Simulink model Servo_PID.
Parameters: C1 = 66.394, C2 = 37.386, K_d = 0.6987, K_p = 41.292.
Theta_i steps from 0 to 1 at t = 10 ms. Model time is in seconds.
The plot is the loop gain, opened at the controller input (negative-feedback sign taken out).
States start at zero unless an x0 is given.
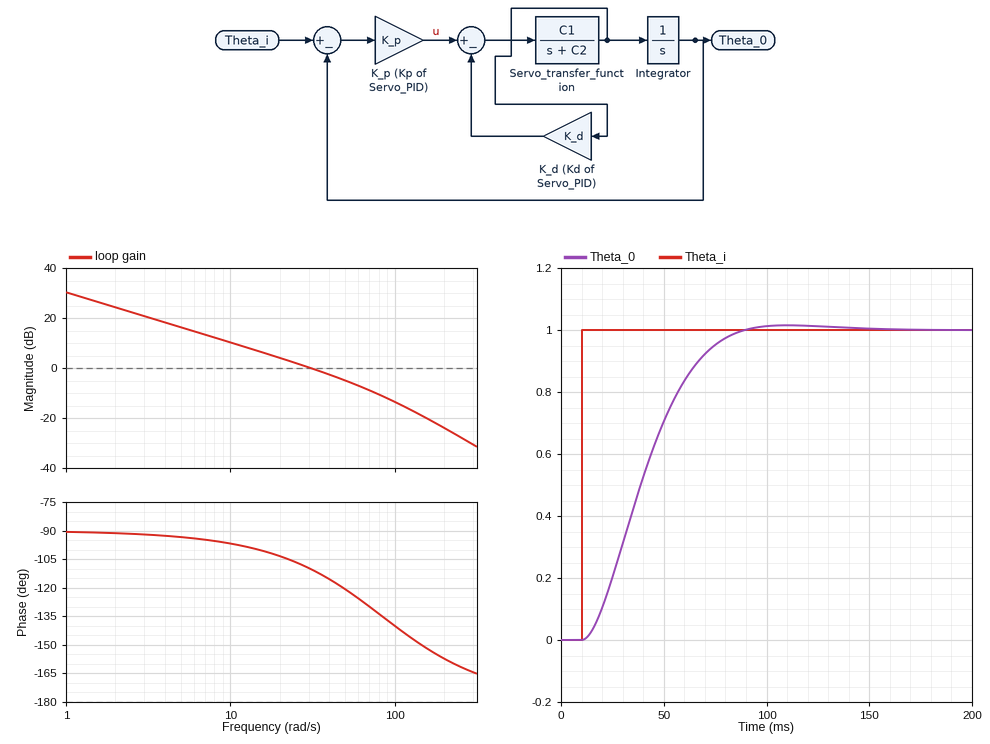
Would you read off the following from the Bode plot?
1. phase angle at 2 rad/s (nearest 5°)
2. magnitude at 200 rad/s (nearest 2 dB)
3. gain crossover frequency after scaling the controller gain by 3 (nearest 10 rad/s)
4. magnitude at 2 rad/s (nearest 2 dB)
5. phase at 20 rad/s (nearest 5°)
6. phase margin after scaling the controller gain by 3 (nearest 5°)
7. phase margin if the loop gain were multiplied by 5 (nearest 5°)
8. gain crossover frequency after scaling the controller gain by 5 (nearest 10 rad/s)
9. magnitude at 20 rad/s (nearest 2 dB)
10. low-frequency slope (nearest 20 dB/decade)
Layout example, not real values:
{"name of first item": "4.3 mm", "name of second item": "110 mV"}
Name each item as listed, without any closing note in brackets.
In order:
{"phase angle at 2 rad/s": "-90°", "magnitude at 200 rad/s": "-24 dB", "gain crossover frequency after scaling the controller gain by 3": "70 rad/s", "magnitude at 2 rad/s": "24 dB", "phase at 20 rad/s": "-105°", "phase margin after scaling the controller gain by 3": "50°", "phase margin if the loop gain were multiplied by 5": "40°", "gain crossover frequency after scaling the controller gain by 5": "100 rad/s", "magnitude at 20 rad/s": "4 dB", "low-frequency slope": "-20 dB/decade"}
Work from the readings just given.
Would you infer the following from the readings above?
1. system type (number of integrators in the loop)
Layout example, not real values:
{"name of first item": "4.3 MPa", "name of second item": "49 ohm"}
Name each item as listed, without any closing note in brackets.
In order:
{"system type": "1"}
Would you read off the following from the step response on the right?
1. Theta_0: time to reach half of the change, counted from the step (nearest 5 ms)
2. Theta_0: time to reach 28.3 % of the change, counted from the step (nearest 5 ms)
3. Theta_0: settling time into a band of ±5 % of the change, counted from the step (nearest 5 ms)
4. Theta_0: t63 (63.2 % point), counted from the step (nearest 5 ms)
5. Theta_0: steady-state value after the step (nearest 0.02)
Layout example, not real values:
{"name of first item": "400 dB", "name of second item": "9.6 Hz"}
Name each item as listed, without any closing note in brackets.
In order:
{"Theta_0: time to reach half of the change, counted from the step": "30 ms", "Theta_0: time to reach 28.3 % of the change, counted from the step": "20 ms", "Theta_0: settling time into a band of ±5 % of the change, counted from the step": "65 ms", "Theta_0: t63 (63.2 % point), counted from the step": "35 ms", "Theta_0: steady-state value after the step": "1.00"}
